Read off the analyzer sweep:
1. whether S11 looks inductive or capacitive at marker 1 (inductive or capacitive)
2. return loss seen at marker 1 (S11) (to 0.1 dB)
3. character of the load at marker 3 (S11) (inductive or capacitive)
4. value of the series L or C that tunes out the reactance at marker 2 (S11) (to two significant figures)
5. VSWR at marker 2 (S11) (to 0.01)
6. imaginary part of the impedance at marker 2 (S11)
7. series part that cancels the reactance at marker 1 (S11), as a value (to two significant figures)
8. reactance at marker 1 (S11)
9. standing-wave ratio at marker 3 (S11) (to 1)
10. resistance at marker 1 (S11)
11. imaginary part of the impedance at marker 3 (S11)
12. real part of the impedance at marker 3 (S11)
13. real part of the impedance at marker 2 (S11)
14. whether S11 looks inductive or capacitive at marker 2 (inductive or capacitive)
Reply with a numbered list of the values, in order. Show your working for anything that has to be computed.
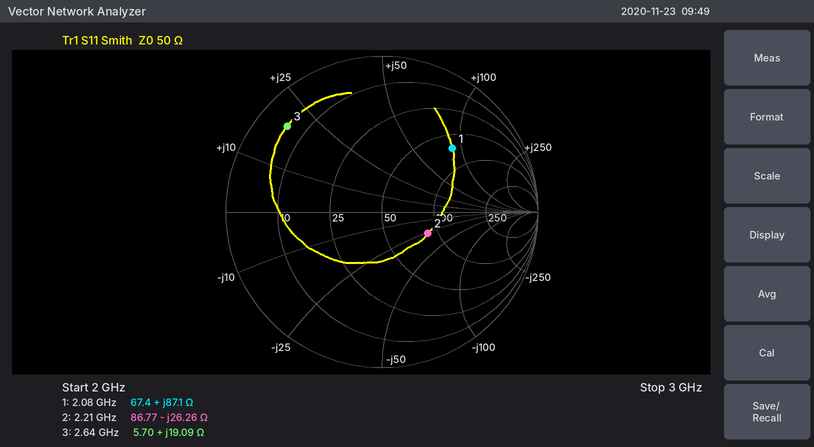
1. inductive
2. 4.3 dB
3. inductive
4. L = 26.26 Ω/(2π × 2.21 GHz) ≈ 1.9 nH
5. 1.96
6. -26.26 Ω
7. C = 1/(2π × 2.08 GHz × 87.1 Ω) ≈ 878 fF, so 880 fF to two significant figures
8. +87.1 Ω
9. 10
10. 67.4 Ω
11. +19.09 Ω
12. 5.70 Ω
13. 86.77 Ω
14. capacitive
